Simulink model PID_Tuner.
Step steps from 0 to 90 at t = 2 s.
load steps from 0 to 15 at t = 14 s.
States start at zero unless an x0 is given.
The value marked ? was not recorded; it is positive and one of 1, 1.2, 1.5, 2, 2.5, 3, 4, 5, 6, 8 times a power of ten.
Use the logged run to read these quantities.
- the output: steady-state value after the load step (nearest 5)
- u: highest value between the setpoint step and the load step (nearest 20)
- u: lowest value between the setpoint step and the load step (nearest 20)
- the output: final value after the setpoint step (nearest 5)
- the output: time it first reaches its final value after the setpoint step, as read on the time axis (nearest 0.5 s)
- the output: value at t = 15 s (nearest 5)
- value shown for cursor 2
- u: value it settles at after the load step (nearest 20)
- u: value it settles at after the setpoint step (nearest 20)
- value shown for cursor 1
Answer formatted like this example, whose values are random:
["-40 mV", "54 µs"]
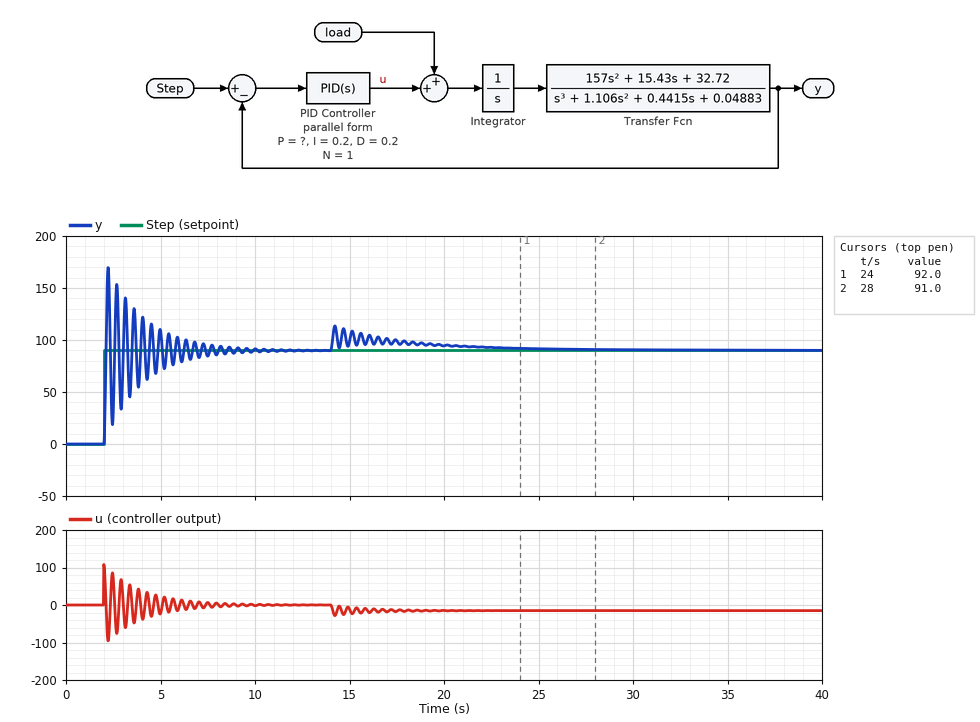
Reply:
["90", "100", "-100", "90", "2.0 s", "100", "91.0", "-20", "0", "92.0"]
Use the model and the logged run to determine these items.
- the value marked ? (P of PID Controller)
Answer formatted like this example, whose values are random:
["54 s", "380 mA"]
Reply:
["1"]
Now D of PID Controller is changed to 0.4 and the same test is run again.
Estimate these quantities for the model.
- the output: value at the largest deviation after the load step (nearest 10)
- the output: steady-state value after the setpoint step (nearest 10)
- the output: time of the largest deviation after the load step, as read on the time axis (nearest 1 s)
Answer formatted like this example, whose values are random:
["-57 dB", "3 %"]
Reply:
["110", "90", "14 s"]
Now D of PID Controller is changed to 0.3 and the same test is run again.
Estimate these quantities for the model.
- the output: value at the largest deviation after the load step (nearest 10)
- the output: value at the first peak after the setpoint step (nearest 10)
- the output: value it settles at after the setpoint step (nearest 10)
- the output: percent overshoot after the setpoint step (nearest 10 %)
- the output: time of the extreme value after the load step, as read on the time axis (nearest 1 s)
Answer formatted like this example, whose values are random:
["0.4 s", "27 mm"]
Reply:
["110", "170", "90", "90 %", "14 s"]
